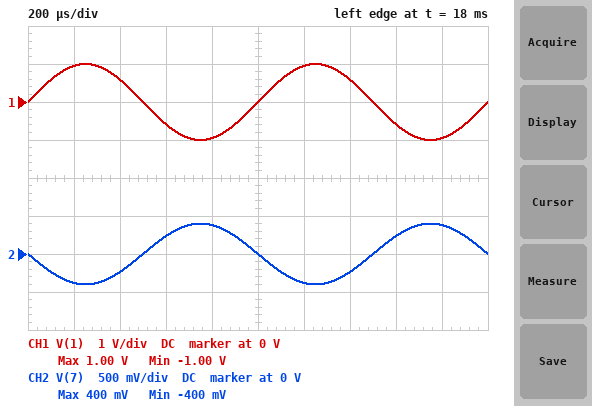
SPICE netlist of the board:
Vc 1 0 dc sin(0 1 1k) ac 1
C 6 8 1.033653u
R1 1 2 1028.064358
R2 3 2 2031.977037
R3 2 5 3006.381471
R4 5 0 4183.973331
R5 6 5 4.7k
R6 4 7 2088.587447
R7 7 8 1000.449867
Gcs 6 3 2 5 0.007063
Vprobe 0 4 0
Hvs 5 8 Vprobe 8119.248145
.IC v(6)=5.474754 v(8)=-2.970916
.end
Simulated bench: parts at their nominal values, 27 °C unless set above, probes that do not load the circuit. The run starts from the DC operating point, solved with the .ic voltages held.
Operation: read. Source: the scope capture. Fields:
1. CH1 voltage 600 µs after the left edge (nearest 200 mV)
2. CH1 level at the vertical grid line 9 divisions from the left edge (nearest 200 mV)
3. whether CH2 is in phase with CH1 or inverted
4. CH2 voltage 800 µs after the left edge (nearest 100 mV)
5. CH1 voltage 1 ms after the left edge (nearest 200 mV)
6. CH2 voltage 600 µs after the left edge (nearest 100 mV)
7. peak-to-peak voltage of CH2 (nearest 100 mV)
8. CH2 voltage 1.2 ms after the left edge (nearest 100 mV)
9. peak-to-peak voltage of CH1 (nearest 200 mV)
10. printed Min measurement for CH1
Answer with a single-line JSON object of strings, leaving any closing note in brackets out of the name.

{"CH1 voltage 600 µs after the left edge": "-600 mV", "CH1 level at the vertical grid line 9 divisions from the left edge": "-1.0 V", "whether CH2 is in phase with CH1 or inverted": "inverted", "CH2 voltage 800 µs after the left edge": "400 mV", "CH1 voltage 1 ms after the left edge": "0 V", "CH2 voltage 600 µs after the left edge": "200 mV", "peak-to-peak voltage of CH2": "800 mV", "CH2 voltage 1.2 ms after the left edge": "-400 mV", "peak-to-peak voltage of CH1": "2.0 V", "printed Min measurement for CH1": "-1.00 V"}
